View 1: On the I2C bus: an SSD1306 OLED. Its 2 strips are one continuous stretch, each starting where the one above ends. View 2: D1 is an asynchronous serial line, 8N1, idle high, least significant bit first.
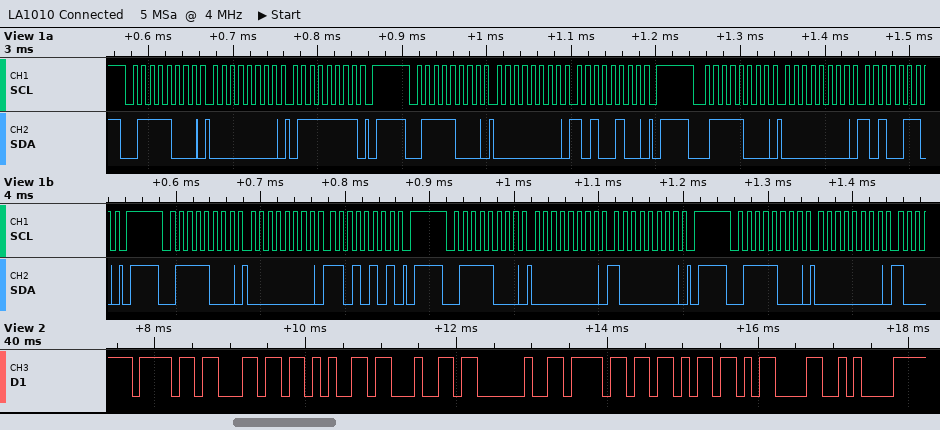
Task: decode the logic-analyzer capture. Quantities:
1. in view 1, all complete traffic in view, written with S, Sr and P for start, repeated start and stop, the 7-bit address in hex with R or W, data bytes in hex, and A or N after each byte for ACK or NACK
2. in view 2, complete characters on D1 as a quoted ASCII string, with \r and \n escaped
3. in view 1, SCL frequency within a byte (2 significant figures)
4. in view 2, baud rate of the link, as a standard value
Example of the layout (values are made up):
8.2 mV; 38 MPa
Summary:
S 3CW A 00 A 7F A P S 3CW A 00 A A4 A P S 3CW A 00 A A6 A P S 3CW A 00 A D5 A P S 3CW A 00 A 80 A P S 3CW A 00 A; "oled ok\r\n"; 100 kHz; 9600 baud
